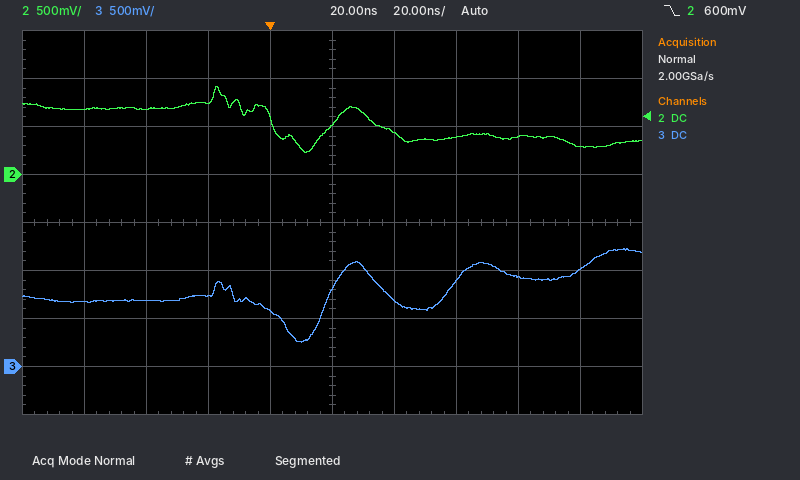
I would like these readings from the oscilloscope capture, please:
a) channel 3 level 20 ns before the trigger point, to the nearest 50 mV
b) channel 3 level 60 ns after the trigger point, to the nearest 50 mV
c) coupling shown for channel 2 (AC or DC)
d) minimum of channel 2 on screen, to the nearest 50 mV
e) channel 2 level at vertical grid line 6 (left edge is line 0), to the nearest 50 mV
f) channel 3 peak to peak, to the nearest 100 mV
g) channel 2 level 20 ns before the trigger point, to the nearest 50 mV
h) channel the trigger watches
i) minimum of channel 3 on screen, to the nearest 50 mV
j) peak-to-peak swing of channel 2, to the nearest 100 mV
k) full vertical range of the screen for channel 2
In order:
750 mV
900 mV
DC
250 mV
450 mV
1.00 V
750 mV
channel 2
250 mV
700 mV
4 V
